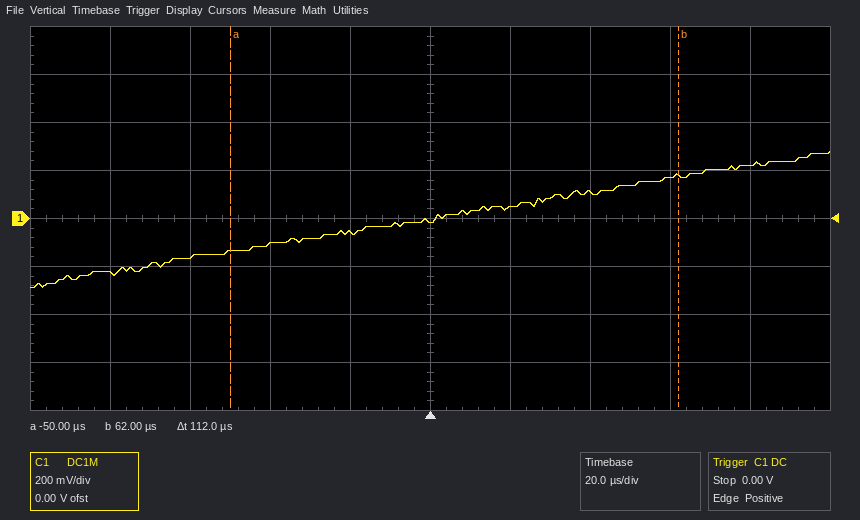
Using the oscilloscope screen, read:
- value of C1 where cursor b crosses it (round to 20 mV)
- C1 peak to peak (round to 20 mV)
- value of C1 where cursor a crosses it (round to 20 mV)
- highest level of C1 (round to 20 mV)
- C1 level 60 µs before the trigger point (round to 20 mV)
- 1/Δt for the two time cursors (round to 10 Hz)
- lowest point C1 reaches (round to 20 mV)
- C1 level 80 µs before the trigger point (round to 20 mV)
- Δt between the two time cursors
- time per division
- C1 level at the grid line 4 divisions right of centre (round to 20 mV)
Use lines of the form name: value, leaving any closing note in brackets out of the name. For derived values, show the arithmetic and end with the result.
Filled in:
value of C1 where cursor b crosses it: 180 mV
C1 peak to peak: 280 mV − (-280 mV) = 560 mV
value of C1 where cursor a crosses it: -140 mV
highest level of C1: 280 mV
C1 level 60 µs before the trigger point: -160 mV
1/Δt for the two time cursors: 1 / 112 µs ≈ 8.93 kHz
lowest point C1 reaches: -280 mV
C1 level 80 µs before the trigger point: -220 mV
Δt between the two time cursors: 112 µs
time per division: 20 µs
C1 level at the grid line 4 divisions right of centre: 220 mV
